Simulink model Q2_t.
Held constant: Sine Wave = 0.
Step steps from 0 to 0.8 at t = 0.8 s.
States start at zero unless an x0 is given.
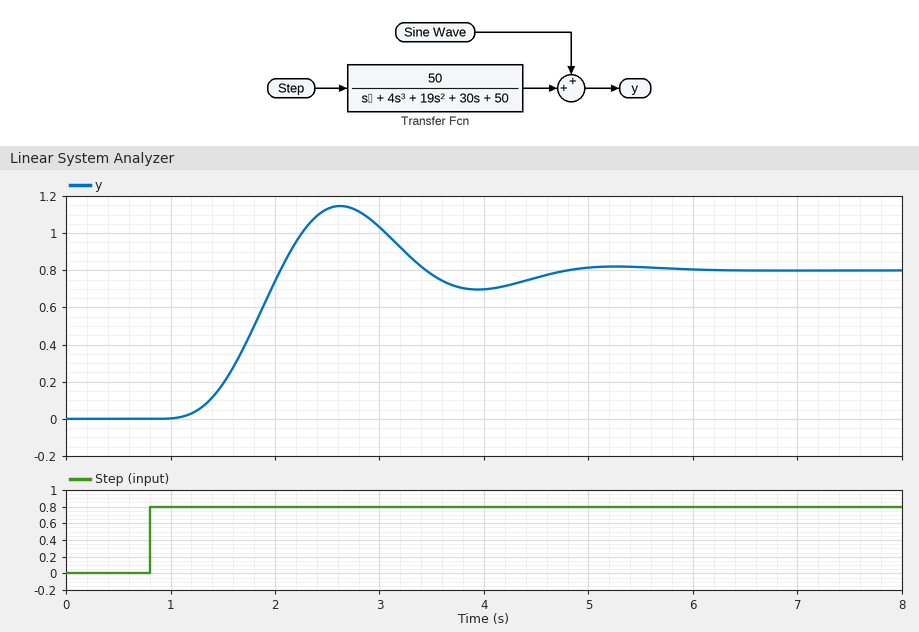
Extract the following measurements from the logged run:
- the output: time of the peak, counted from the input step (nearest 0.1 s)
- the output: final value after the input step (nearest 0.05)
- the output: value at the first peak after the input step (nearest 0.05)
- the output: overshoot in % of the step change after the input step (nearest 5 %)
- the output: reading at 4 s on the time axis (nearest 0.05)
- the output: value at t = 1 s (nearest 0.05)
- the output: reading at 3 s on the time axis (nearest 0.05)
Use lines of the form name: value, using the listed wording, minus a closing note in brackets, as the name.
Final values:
the output: time of the peak, counted from the input step: 1.8 s
the output: final value after the input step: 0.80
the output: value at the first peak after the input step: 1.15
the output: overshoot in % of the step change after the input step: 45 %
the output: reading at 4 s on the time axis: 0.70
the output: value at t = 1 s: 0.00
the output: reading at 3 s on the time axis: 1.05
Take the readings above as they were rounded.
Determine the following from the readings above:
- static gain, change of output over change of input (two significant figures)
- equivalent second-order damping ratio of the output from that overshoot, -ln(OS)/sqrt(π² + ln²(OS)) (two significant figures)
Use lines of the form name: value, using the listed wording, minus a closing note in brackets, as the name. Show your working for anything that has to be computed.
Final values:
static gain, change of output over change of input: (0.8 - 0) / (0.8 - 0) = 1.0
equivalent second-order damping ratio of the output from that overshoot, -ln(OS)/sqrt(π² + ln²(OS)): ln(0.45) = -0.799; 0.799 / sqrt(9.870 + 0.638) = 0.25
